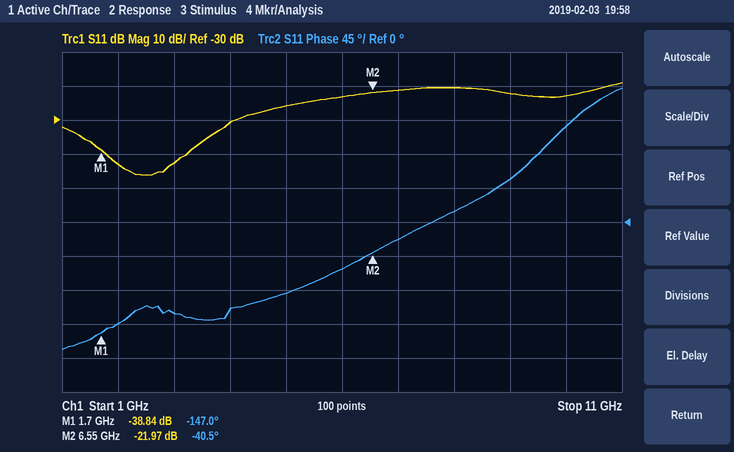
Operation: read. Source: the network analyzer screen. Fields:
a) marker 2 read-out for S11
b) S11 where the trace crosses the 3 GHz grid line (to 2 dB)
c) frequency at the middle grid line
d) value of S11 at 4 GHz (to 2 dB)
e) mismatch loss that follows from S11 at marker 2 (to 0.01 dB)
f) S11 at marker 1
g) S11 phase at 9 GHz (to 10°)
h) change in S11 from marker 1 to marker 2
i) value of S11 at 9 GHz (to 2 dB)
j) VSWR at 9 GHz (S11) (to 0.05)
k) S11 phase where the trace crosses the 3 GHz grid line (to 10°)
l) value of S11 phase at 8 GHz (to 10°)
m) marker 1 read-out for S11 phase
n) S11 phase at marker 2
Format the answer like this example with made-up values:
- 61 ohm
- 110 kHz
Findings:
- -21.97 dB
- -42 dB
- 6 GHz
- -30 dB
- 0.03 dB
- -38.84 dB
- 60°
- 16.87 dB
- -22 dB
- 1.15
- -120°
- 10°
- -147.0°
- -40.5°
